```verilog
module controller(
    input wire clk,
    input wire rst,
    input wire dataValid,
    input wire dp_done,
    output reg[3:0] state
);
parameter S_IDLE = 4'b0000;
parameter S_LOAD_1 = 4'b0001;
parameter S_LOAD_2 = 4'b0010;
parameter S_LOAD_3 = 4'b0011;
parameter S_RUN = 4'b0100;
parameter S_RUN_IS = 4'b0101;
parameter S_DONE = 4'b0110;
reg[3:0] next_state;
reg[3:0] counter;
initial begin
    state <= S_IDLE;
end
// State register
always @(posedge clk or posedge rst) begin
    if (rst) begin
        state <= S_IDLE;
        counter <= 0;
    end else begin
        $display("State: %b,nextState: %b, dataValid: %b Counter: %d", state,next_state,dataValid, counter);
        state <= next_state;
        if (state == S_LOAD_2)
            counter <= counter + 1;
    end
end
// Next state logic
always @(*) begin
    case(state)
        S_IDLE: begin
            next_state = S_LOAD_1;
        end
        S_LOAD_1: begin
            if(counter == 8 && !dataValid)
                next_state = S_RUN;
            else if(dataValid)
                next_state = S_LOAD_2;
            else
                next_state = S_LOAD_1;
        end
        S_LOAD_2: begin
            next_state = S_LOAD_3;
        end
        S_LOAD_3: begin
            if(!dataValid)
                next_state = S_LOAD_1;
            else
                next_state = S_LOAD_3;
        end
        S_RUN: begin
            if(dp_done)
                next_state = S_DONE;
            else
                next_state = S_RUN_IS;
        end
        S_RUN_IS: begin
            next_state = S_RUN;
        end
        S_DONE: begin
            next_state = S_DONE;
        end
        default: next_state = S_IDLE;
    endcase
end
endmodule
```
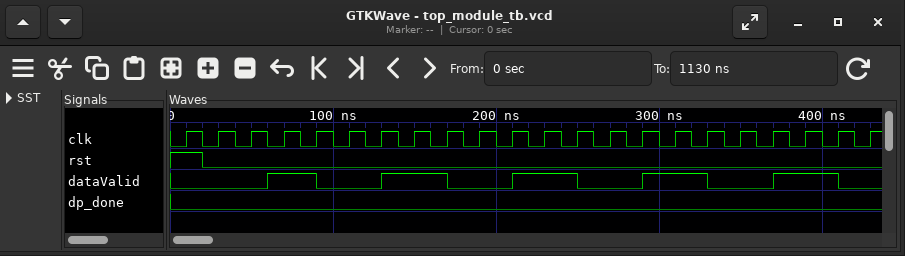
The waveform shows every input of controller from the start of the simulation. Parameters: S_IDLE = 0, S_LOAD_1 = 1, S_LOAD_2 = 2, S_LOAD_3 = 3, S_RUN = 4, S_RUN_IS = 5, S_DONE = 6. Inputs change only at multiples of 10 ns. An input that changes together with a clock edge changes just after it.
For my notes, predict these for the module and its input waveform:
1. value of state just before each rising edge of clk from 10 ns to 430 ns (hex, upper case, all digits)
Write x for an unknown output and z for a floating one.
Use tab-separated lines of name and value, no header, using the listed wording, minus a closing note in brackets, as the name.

value of state just before each rising edge of clk from 10 ns to 430 ns	0, 0, 1, 1, 2, 3, 1, 1, 2, 3, 1, 1, 2, 3, 1, 1, 2, 3, 1, 1, 2, 3
